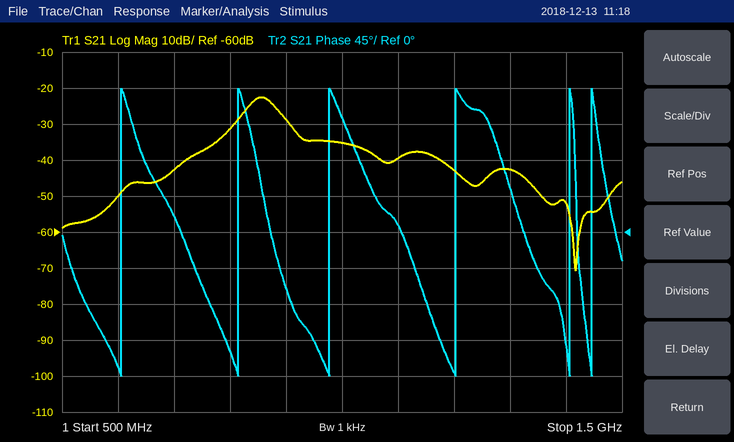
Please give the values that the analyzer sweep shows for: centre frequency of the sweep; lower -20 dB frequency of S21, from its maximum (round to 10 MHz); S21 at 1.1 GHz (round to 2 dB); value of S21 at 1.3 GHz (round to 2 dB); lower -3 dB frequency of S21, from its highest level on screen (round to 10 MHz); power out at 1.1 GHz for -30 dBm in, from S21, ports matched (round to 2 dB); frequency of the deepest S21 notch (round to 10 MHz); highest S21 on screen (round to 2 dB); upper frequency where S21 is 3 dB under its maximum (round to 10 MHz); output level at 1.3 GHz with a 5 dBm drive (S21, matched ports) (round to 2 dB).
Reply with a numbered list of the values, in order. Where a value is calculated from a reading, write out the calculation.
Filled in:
1. 1 GHz
2. 700 MHz
3. -40 dB
4. -42 dB
5. 830 MHz
6. -30 dBm + (-40 dB) = -70 dBm
7. 1.42 GHz
8. -22 dB
9. 880 MHz
10. 5 dBm + (-42 dB) = -38 dBm
